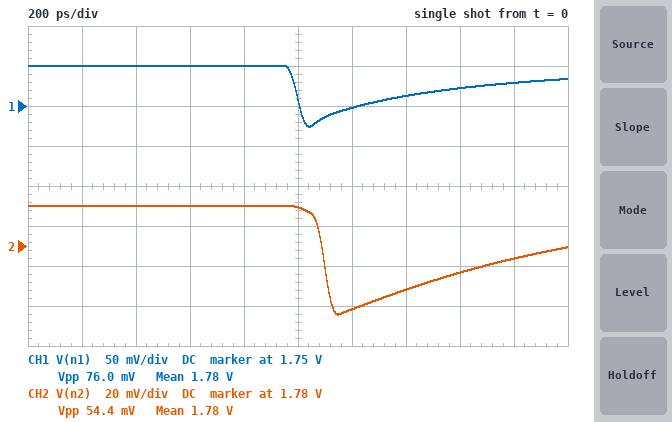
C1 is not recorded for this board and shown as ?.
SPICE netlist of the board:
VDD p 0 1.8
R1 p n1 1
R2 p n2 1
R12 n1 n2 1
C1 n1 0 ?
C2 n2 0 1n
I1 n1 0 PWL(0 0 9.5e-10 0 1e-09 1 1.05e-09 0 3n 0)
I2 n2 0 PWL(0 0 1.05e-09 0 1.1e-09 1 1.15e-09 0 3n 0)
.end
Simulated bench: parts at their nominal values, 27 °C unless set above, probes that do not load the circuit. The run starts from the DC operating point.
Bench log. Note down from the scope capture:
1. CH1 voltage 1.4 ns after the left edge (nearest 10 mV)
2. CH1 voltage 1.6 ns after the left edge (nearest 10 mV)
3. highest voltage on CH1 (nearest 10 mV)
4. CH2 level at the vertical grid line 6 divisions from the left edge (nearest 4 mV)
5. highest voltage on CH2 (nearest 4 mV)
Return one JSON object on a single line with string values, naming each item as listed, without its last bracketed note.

{"CH1 voltage 1.4 ns after the left edge": "1.76 V", "CH1 voltage 1.6 ns after the left edge": "1.77 V", "highest voltage on CH1": "1.80 V", "CH2 level at the vertical grid line 6 divisions from the left edge": "1.748 V", "highest voltage on CH2": "1.800 V"}
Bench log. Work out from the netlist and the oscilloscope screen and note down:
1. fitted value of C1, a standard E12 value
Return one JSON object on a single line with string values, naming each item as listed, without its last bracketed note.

{"fitted value of C1, a standard E12 value": "560 pF"}
